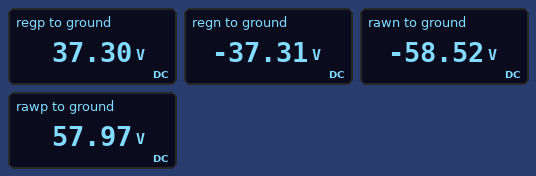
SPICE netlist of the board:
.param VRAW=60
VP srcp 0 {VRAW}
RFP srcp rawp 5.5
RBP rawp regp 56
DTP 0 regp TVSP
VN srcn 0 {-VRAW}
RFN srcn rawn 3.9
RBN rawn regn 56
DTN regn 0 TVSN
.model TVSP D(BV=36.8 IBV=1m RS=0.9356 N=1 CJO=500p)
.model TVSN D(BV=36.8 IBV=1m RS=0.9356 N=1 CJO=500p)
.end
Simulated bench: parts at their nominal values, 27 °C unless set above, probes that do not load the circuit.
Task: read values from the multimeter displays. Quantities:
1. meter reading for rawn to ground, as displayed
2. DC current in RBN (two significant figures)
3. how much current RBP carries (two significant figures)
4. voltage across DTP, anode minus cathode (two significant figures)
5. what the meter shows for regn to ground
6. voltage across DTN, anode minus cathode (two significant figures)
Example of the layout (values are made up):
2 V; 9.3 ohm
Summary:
-58.52 V; 380 mA; 370 mA; -37 V; -37.31 V; -37 V
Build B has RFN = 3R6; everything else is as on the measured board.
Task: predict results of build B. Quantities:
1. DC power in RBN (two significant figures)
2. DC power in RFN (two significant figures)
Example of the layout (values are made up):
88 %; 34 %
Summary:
8.1 W; 520 mW
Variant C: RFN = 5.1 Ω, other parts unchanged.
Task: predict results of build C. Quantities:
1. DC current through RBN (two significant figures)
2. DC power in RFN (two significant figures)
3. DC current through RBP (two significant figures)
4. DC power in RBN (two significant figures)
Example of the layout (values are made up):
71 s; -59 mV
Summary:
370 mA; 700 mW; 370 mA; 7.7 W
